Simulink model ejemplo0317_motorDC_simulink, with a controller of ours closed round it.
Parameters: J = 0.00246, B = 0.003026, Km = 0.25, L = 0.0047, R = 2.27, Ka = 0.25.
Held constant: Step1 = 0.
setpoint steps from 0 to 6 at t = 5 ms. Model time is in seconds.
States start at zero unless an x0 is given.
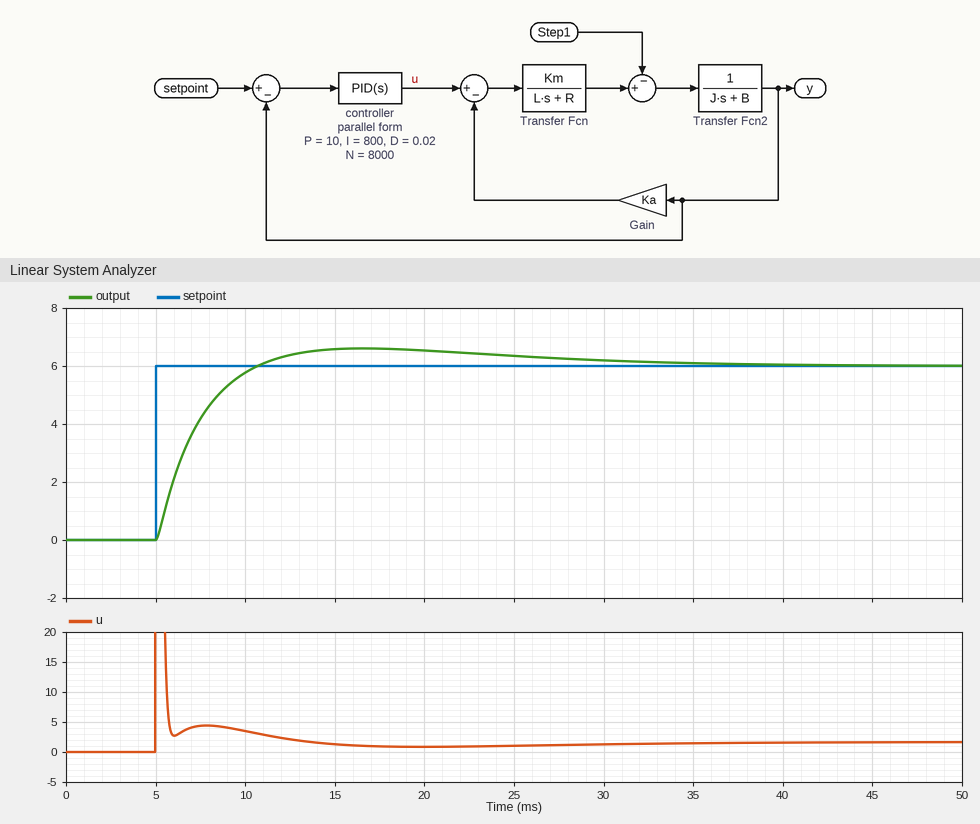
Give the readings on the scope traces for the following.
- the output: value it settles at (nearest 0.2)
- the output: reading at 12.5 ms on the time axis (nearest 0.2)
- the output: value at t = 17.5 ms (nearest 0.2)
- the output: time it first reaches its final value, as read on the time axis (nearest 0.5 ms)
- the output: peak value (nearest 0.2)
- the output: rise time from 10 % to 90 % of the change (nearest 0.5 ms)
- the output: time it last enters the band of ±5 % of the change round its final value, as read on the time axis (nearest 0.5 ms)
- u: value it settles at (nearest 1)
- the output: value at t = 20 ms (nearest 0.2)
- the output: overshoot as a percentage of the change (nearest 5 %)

6.0
6.4
6.6
10.5 ms
6.6
4.0 ms
26.5 ms
2
6.6
10 %
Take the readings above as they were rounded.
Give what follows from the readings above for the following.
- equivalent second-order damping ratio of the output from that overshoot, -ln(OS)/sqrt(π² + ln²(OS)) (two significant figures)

0.59
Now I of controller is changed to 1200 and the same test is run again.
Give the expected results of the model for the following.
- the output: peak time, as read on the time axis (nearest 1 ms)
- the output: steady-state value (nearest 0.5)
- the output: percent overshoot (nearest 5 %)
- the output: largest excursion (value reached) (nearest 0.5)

15 ms
6.0
15 %
7.0
